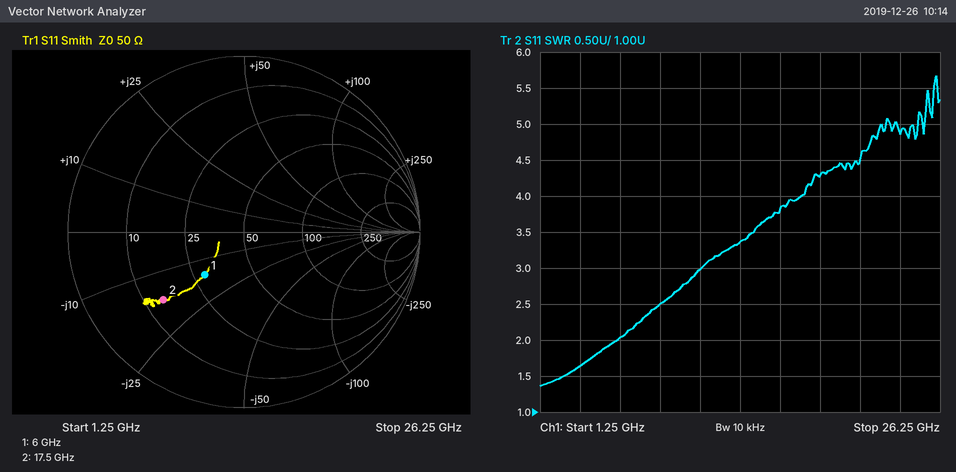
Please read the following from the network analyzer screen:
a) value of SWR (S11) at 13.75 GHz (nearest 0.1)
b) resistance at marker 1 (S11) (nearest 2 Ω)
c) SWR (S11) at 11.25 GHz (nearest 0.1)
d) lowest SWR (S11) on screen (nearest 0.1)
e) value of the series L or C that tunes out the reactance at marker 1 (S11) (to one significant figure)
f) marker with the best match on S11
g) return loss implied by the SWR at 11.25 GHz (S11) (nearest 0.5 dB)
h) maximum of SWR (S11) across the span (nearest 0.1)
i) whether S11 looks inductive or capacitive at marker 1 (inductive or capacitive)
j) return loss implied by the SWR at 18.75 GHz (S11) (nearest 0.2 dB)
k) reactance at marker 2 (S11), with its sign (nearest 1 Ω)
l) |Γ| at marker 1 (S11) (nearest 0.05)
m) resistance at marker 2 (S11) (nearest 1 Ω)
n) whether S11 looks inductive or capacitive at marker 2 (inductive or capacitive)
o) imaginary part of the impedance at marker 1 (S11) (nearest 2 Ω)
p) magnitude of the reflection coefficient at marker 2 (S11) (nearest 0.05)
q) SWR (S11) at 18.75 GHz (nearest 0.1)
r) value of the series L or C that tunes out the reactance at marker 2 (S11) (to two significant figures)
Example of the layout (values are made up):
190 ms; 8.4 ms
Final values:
3.4; 28 Ω; 3.0; 1.4; 400 pH; marker 1; 6.0 dB; 5.7; capacitive; 4.2 dB; -17 Ω; 0.35; 14 Ω; capacitive; -16 Ω; 0.60; 4.3; 150 pH
